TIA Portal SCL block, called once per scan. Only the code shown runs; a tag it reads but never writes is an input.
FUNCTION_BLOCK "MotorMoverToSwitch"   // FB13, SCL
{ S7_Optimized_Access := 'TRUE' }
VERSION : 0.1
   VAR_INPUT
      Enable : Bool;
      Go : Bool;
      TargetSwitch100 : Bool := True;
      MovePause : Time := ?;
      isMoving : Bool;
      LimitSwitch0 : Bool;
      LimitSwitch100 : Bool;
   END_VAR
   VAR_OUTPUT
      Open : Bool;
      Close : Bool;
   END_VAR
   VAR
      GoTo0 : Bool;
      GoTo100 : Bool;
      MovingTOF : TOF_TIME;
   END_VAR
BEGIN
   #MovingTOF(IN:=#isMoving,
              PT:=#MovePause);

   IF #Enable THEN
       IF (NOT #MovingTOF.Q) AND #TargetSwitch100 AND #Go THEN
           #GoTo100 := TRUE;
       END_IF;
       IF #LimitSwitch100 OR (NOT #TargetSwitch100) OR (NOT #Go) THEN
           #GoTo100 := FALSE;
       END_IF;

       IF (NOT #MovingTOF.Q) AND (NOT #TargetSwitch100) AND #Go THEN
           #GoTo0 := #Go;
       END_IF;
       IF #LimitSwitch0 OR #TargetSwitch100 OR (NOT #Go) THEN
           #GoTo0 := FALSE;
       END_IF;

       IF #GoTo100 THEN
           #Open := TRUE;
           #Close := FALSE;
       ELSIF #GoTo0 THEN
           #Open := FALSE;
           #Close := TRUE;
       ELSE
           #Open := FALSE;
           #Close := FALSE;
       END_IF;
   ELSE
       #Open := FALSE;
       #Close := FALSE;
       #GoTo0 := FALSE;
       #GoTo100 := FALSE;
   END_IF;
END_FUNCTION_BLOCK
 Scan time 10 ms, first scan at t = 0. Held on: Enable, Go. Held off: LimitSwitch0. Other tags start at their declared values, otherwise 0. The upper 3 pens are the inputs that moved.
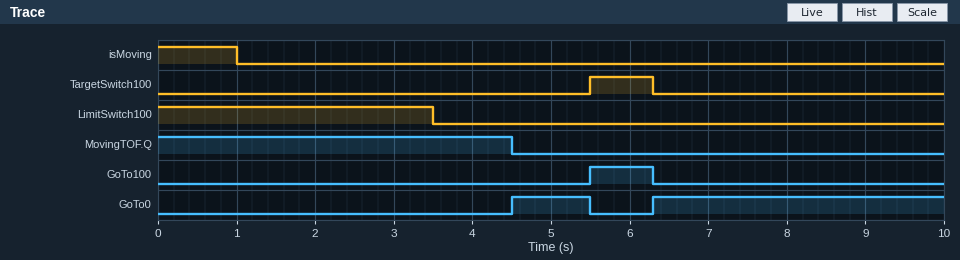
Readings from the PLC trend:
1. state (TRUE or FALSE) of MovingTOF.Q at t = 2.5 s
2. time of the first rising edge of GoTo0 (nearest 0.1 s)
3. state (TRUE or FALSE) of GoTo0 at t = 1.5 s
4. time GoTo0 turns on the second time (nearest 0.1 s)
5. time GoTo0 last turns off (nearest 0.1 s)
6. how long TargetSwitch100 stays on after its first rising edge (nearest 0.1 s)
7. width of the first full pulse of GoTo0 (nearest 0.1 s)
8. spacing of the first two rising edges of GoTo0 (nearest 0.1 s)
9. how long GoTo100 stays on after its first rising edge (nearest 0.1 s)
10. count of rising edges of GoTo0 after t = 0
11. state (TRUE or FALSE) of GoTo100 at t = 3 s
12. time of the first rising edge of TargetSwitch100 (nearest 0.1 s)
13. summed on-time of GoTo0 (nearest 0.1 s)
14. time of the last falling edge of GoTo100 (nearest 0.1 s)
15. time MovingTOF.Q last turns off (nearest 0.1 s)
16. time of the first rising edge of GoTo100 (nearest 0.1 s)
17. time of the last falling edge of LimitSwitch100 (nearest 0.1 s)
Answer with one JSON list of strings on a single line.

["TRUE", "4.5 s", "FALSE", "6.3 s", "5.5 s", "0.8 s", "1.0 s", "1.8 s", "0.8 s", "2", "FALSE", "5.5 s", "4.7 s", "6.3 s", "4.5 s", "5.5 s", "3.5 s"]
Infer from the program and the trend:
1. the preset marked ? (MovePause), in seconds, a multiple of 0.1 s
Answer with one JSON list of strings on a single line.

["3.5 s"]
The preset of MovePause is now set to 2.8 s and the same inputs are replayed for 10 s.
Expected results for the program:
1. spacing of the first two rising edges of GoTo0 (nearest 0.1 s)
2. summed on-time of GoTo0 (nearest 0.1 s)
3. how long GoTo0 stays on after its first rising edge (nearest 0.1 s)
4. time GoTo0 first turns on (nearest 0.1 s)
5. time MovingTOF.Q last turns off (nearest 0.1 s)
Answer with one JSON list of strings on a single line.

["2.5 s", "5.4 s", "1.7 s", "3.8 s", "3.8 s"]
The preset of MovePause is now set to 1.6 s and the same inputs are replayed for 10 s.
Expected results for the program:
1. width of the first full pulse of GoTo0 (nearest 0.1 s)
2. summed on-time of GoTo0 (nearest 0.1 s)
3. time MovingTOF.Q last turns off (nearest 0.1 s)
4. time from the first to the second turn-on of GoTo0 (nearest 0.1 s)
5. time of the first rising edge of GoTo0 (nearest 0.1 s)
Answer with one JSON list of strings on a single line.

["2.9 s", "6.6 s", "2.6 s", "3.7 s", "2.6 s"]
